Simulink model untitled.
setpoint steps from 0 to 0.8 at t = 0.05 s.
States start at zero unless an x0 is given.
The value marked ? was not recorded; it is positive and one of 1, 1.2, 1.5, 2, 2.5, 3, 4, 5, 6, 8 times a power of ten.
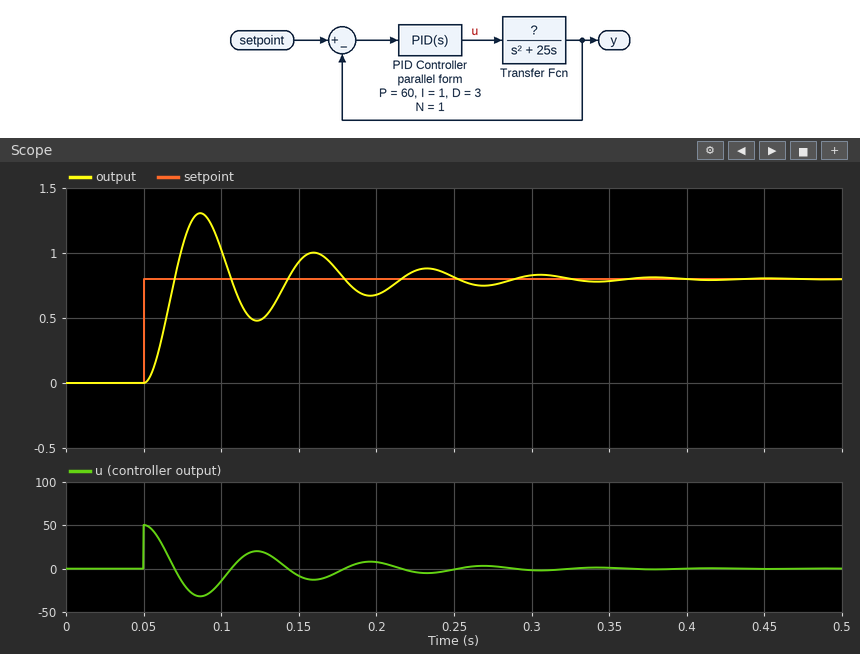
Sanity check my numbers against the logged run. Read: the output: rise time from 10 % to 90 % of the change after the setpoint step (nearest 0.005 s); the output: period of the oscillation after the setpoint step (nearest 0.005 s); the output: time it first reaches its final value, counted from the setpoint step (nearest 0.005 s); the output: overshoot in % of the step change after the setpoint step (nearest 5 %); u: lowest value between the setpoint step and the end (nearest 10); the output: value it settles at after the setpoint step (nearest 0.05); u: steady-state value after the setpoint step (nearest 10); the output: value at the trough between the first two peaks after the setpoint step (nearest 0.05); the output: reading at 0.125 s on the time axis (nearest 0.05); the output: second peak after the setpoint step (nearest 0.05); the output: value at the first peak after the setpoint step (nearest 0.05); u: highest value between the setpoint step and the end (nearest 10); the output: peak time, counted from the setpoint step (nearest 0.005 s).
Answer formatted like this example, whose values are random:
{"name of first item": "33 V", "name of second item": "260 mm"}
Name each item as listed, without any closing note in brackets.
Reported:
{"the output: rise time from 10 % to 90 % of the change after the setpoint step": "0.015 s", "the output: period of the oscillation after the setpoint step": "0.075 s", "the output: time it first reaches its final value, counted from the setpoint step": "0.020 s", "the output: overshoot in % of the step change after the setpoint step": "65 %", "u: lowest value between the setpoint step and the end": "-30", "the output: value it settles at after the setpoint step": "0.80", "u: steady-state value after the setpoint step": "0", "the output: value at the trough between the first two peaks after the setpoint step": "0.50", "the output: reading at 0.125 s on the time axis": "0.50", "the output: second peak after the setpoint step": "1.00", "the output: value at the first peak after the setpoint step": "1.30", "u: highest value between the setpoint step and the end": "50", "the output: peak time, counted from the setpoint step": "0.035 s"}
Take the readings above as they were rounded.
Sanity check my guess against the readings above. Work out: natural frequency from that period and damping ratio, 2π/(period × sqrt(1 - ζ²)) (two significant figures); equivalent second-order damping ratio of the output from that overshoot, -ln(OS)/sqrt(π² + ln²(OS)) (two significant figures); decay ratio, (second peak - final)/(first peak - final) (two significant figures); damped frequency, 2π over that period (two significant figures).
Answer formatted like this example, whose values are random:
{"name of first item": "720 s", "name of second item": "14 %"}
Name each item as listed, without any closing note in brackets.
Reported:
{"natural frequency from that period and damping ratio, 2π/(period × sqrt(1 - ζ²))": "85 rad/s", "equivalent second-order damping ratio of the output from that overshoot, -ln(OS)/sqrt(π² + ln²(OS))": "0.14", "decay ratio, (second peak - final)/(first peak - final)": "0.40", "damped frequency, 2π over that period": "84 rad/s"}
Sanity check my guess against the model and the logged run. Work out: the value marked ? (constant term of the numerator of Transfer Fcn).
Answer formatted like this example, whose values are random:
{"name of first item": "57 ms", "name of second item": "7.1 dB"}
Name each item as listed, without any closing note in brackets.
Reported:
{"the value marked ?": "120"}
